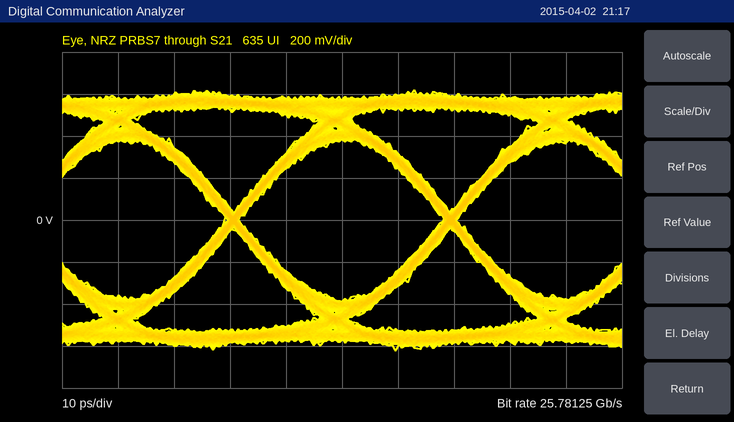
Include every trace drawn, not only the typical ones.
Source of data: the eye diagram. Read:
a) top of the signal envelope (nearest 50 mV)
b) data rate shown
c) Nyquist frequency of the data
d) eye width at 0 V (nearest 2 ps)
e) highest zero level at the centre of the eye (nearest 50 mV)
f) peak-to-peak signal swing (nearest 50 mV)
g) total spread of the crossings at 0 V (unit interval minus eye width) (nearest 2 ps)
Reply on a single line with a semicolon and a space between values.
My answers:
600 mV; 25.78125 Gb/s; 12.89062 GHz; 36 ps; -400 mV; 1.25 V; 2 ps
